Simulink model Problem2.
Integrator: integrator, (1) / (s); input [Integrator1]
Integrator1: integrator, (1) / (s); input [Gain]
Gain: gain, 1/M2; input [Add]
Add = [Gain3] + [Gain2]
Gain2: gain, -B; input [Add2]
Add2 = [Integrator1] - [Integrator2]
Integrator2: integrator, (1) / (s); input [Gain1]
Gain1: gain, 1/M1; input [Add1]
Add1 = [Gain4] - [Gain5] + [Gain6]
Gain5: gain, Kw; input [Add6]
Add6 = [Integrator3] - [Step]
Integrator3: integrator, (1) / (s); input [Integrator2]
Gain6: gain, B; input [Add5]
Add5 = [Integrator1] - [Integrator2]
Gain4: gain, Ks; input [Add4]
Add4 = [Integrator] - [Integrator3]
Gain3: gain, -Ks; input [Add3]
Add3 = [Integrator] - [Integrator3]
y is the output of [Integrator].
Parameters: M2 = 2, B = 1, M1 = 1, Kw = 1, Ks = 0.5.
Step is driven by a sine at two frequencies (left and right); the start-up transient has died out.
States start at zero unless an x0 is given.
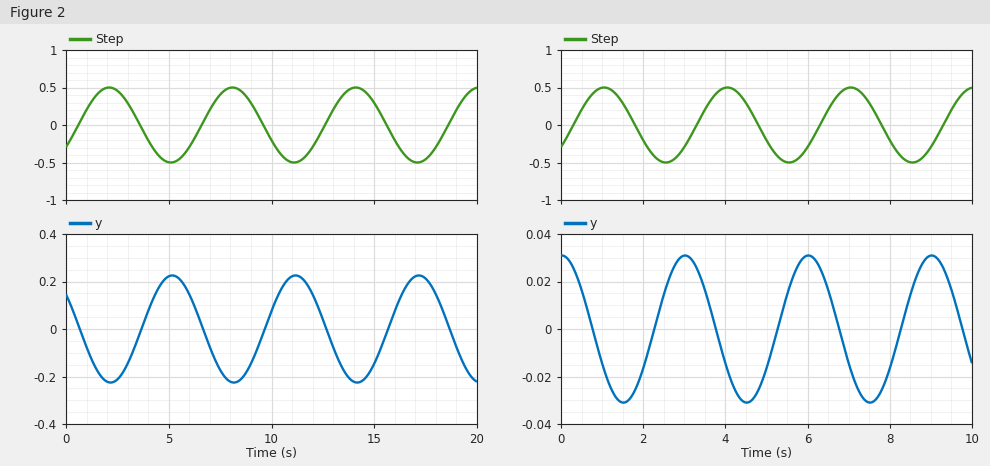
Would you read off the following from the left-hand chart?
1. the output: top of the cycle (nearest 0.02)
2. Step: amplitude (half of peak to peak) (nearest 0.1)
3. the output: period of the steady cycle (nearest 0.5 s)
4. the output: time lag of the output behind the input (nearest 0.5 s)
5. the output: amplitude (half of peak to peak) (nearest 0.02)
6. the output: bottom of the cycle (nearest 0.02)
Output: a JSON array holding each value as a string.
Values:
["0.22", "0.5", "6.0 s", "3.0 s", "0.22", "-0.22"]
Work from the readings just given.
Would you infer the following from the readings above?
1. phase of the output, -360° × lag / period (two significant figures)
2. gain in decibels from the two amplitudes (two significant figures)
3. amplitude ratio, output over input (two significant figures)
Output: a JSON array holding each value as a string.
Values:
["-180°", "-7.1 dB", "0.44"]
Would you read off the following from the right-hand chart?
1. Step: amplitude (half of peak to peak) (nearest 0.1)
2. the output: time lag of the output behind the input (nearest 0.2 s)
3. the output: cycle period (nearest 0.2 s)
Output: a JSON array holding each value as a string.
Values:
["0.5", "2.0 s", "3.0 s"]
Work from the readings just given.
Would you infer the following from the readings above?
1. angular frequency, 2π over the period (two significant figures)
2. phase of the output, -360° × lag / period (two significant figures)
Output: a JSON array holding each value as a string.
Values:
["2.1 rad/s", "-240°"]
